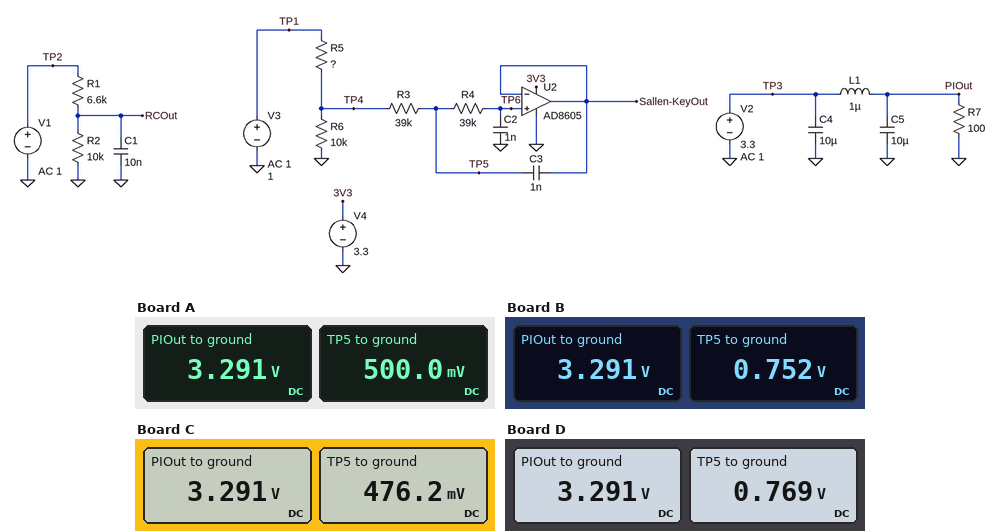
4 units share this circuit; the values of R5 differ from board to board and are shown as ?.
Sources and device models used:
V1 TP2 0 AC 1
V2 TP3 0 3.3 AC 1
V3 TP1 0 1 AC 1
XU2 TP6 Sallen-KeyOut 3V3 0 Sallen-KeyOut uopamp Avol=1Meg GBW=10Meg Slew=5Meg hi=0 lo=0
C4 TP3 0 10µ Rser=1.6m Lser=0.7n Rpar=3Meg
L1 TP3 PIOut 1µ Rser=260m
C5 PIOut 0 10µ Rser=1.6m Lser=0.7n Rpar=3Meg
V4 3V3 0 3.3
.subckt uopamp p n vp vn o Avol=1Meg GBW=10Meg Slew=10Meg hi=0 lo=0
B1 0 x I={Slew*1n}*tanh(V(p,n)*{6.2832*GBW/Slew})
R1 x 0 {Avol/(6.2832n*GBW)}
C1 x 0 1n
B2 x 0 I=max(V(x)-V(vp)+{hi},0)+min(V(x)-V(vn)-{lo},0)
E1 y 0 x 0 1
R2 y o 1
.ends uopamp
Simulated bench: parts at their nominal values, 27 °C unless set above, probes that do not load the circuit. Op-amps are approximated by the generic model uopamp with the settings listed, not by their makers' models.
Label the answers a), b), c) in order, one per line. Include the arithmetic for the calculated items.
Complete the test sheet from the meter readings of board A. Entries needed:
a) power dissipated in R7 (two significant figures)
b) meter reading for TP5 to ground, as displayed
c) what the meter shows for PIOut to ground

a) (3.291 V)^2 / 100 Ω = 110 mW
b) 500.0 mV
c) 3.291 V
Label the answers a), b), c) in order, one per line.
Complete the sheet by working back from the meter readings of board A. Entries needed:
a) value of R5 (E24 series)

a) 10 kΩ
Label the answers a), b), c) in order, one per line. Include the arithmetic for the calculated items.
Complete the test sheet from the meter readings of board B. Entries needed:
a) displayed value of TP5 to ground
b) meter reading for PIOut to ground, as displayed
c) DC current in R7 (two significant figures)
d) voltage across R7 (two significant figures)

a) 0.752 V
b) 3.291 V
c) (3.291 V) / 100 Ω = 33 mA
d) 3.291 V = 3.3 V
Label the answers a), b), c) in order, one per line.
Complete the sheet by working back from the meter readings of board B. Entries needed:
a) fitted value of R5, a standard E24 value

a) 3.3 kΩ
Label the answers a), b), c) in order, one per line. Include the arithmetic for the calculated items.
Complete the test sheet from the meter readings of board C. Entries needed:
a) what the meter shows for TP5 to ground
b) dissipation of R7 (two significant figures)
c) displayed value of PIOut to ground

a) 476.2 mV
b) (3.291 V)^2 / 100 Ω = 110 mW
c) 3.291 V
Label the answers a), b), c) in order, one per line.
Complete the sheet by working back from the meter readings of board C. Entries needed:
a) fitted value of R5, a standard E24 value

a) 11 kΩ
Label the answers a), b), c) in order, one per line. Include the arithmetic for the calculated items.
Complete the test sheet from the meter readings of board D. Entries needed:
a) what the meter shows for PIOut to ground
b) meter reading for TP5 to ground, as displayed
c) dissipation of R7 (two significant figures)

a) 3.291 V
b) 0.769 V
c) (3.291 V)^2 / 100 Ω = 110 mW
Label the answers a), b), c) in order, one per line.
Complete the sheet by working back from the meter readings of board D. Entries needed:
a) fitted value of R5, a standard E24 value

a) 3 kΩ
